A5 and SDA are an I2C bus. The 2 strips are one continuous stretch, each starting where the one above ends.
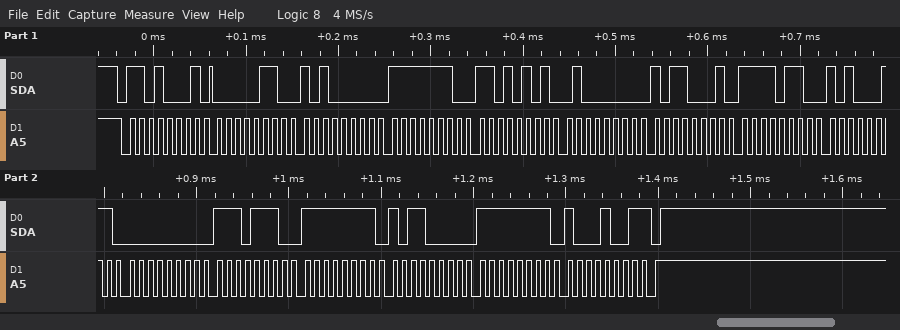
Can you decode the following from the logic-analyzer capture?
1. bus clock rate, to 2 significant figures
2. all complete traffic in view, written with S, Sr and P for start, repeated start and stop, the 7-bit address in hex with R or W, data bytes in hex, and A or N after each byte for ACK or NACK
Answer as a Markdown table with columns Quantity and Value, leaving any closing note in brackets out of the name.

| Quantity | Value |
|---|---|
| bus clock rate, to 2 significant figures | 100 kHz |
| all complete traffic in view, written with S, Sr and P for start, repeated start and stop, the 7-bit address in hex with R or W, data bytes in hex, and A or N after each byte for ACK or NACK | S 68R A 06 A A0 A FE A D5 A 40 A B1 A F6 A A3 A 00 A EE A FF A B0 A FF A 89 N P |
